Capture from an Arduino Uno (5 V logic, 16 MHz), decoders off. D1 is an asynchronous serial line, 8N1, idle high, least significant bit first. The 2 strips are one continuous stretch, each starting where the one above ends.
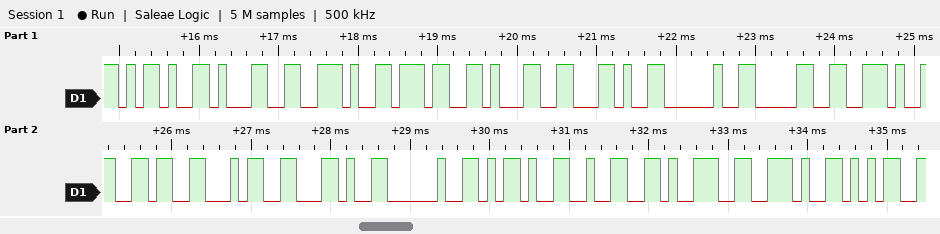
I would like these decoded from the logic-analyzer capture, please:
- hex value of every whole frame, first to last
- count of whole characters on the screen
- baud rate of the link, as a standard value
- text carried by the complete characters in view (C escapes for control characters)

0x2D 0x31 0x2E 0x37 0x31 0x2C 0x20 0x30 0x2E 0x36 0x34 0x2C 0x20 0x2D 0x32 0x39 0x2E 0x35
18
9600 baud
"-1.71, 0.64, -29.5"
